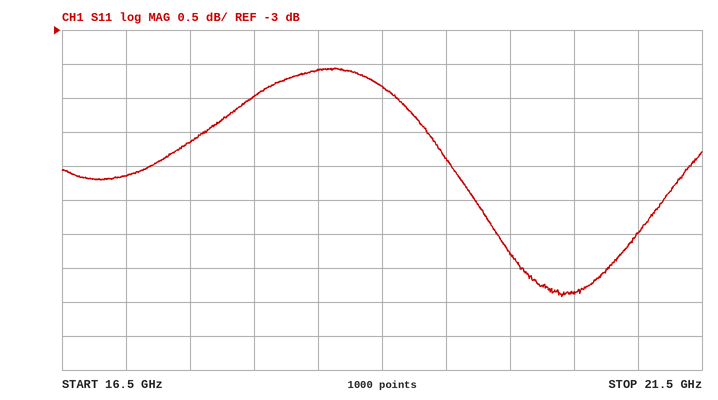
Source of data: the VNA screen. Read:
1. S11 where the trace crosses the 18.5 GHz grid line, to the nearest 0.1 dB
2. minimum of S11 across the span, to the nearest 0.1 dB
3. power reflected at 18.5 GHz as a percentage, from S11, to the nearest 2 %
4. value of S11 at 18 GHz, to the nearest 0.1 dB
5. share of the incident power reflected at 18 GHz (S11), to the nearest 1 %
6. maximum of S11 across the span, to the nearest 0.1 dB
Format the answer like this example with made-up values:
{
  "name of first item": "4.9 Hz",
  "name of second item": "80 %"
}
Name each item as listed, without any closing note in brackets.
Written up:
{
  "S11 where the trace crosses the 18.5 GHz grid line, to the nearest 0.1 dB": "-3.6 dB",
  "minimum of S11 across the span, to the nearest 0.1 dB": "-6.9 dB",
  "power reflected at 18.5 GHz as a percentage, from S11, to the nearest 2 %": "44 %",
  "value of S11 at 18 GHz, to the nearest 0.1 dB": "-4.0 dB",
  "share of the incident power reflected at 18 GHz (S11), to the nearest 1 %": "40 %",
  "maximum of S11 across the span, to the nearest 0.1 dB": "-3.6 dB"
}
